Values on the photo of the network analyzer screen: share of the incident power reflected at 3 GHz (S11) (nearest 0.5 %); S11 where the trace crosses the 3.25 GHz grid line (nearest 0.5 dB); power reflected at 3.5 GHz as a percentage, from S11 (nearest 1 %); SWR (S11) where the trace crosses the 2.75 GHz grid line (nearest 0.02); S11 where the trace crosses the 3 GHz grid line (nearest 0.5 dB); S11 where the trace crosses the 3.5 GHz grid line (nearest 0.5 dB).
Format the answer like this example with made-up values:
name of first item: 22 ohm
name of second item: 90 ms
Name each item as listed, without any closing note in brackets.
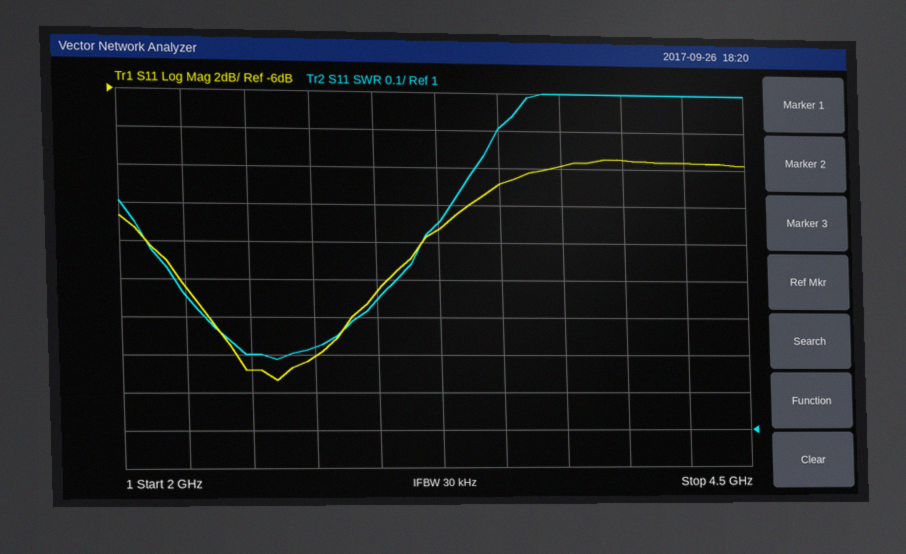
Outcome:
share of the incident power reflected at 3 GHz (S11): 2.0 %
S11 where the trace crosses the 3.25 GHz grid line: -13.5 dB
power reflected at 3.5 GHz as a percentage, from S11: 8 %
SWR (S11) where the trace crosses the 2.75 GHz grid line: 1.22
S11 where the trace crosses the 3 GHz grid line: -16.5 dB
S11 where the trace crosses the 3.5 GHz grid line: -11.0 dB
